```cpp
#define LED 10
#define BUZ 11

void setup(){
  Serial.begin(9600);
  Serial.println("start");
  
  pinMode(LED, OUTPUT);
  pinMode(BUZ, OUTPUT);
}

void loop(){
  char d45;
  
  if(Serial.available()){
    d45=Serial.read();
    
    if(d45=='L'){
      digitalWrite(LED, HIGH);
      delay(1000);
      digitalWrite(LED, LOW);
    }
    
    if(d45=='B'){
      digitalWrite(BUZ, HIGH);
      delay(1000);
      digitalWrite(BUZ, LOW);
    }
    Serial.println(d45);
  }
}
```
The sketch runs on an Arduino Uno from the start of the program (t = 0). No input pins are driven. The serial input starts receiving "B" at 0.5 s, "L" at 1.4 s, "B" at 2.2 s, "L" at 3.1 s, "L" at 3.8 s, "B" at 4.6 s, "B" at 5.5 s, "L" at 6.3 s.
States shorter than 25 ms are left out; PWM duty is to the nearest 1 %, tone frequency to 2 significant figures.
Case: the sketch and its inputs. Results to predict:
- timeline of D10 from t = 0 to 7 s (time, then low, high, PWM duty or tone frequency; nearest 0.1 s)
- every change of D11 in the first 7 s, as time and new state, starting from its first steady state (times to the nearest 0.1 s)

0 s low; 1.5 s high; 2.5 s low; 3.5 s high; 5.5 s low
0 s low; 0.5 s high; 1.5 s low; 2.5 s high; 3.5 s low; 5.5 s high
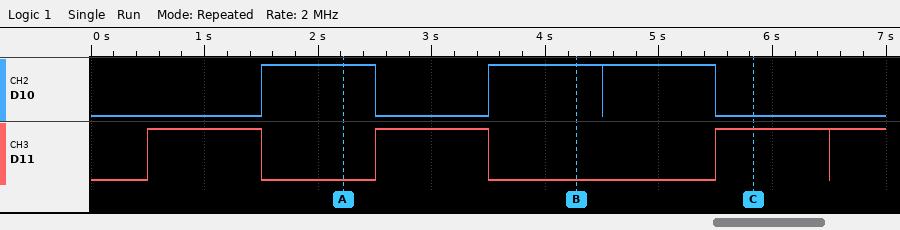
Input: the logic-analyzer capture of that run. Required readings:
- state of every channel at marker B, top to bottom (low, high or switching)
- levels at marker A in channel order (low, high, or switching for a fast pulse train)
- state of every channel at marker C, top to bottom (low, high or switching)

D10 high, D11 low
D10 high, D11 low
D10 low, D11 high
